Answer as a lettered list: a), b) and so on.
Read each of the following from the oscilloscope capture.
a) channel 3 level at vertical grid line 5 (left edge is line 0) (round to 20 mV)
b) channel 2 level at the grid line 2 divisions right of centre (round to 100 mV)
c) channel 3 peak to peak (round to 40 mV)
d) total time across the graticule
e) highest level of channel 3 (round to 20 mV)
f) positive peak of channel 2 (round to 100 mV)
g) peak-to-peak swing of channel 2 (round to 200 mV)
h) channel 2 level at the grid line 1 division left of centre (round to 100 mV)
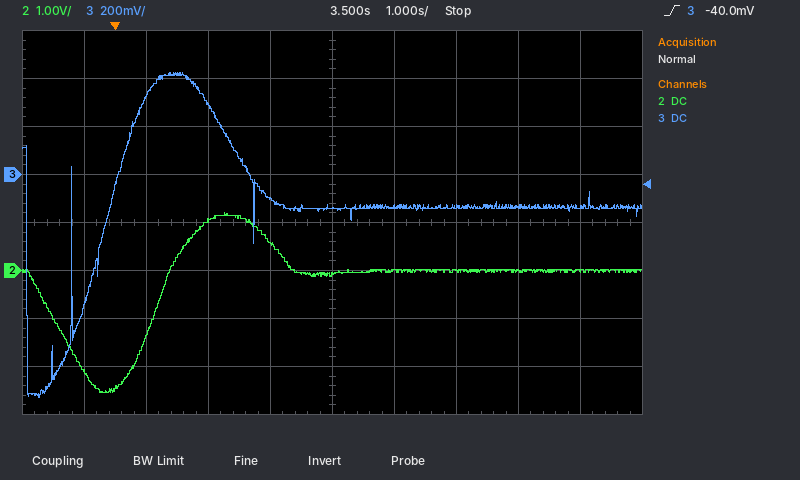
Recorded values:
a) -140 mV
b) 0.0 V
c) 1.36 V
d) 10 s
e) 420 mV
f) 1.2 V
g) 3.8 V
h) 600 mV
